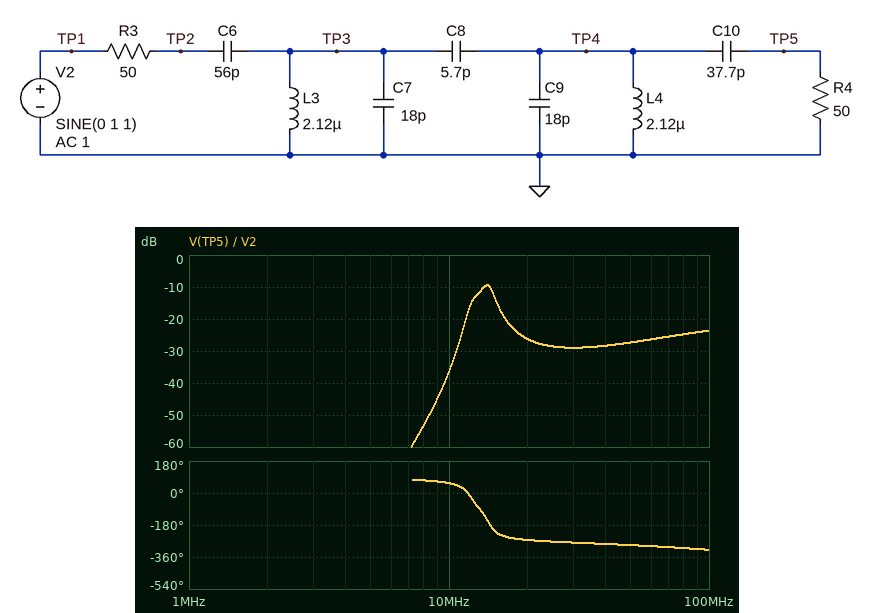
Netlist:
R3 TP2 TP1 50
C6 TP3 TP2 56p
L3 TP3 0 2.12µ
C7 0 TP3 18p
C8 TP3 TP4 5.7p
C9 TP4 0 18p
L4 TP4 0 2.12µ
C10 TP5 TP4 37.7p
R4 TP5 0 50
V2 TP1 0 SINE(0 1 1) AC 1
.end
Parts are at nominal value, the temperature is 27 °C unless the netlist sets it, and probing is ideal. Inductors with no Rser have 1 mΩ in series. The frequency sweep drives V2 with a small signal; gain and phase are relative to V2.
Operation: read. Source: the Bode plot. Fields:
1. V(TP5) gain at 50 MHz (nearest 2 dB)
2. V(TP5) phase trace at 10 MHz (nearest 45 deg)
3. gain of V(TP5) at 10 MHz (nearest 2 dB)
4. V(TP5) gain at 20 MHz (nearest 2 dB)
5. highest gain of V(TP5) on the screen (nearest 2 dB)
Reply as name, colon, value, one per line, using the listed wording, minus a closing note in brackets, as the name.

V(TP5) gain at 50 MHz: -28 dB
V(TP5) phase trace at 10 MHz: 45 deg
gain of V(TP5) at 10 MHz: -36 dB
V(TP5) gain at 20 MHz: -26 dB
highest gain of V(TP5) on the screen: -10 dB
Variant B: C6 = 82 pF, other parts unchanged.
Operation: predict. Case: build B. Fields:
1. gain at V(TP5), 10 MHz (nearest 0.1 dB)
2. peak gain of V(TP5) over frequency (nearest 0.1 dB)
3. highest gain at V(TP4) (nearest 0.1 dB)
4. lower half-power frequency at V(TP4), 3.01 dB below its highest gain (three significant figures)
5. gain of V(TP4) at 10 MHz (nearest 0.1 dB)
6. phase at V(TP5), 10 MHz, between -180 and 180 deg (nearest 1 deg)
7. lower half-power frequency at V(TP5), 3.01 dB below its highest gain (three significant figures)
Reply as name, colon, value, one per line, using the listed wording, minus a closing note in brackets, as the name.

gain at V(TP5), 10 MHz: -29.5 dB
peak gain of V(TP5) over frequency: -12.1 dB
highest gain at V(TP4): 3.6 dB
lower half-power frequency at V(TP4), 3.01 dB below its highest gain: 13.2 MHz
gain of V(TP4) at 10 MHz: -10.9 dB
phase at V(TP5), 10 MHz, between -180 and 180 deg: 17 deg
lower half-power frequency at V(TP5), 3.01 dB below its highest gain: 13.3 MHz
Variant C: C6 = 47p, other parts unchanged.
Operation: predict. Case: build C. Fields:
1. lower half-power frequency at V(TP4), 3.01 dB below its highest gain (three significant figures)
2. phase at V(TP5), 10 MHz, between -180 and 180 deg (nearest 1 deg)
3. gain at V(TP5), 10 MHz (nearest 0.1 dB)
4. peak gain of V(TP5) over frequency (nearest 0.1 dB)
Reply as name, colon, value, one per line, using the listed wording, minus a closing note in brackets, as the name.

lower half-power frequency at V(TP4), 3.01 dB below its highest gain: 12.7 MHz
phase at V(TP5), 10 MHz, between -180 and 180 deg: 63 deg
gain at V(TP5), 10 MHz: -39.4 dB
peak gain of V(TP5) over frequency: -7.6 dB
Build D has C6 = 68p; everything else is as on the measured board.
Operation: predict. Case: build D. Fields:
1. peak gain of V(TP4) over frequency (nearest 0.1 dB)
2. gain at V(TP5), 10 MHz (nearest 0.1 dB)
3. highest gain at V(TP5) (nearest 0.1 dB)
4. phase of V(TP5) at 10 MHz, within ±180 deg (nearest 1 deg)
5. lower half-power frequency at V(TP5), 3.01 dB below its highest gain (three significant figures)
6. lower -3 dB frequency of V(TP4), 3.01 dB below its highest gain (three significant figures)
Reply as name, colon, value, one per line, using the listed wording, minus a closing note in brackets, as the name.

peak gain of V(TP4) over frequency: 4.8 dB
gain at V(TP5), 10 MHz: -32.8 dB
highest gain at V(TP5): -10.9 dB
phase of V(TP5) at 10 MHz, within ±180 deg: 42 deg
lower half-power frequency at V(TP5), 3.01 dB below its highest gain: 13.2 MHz
lower -3 dB frequency of V(TP4), 3.01 dB below its highest gain: 13.0 MHz
